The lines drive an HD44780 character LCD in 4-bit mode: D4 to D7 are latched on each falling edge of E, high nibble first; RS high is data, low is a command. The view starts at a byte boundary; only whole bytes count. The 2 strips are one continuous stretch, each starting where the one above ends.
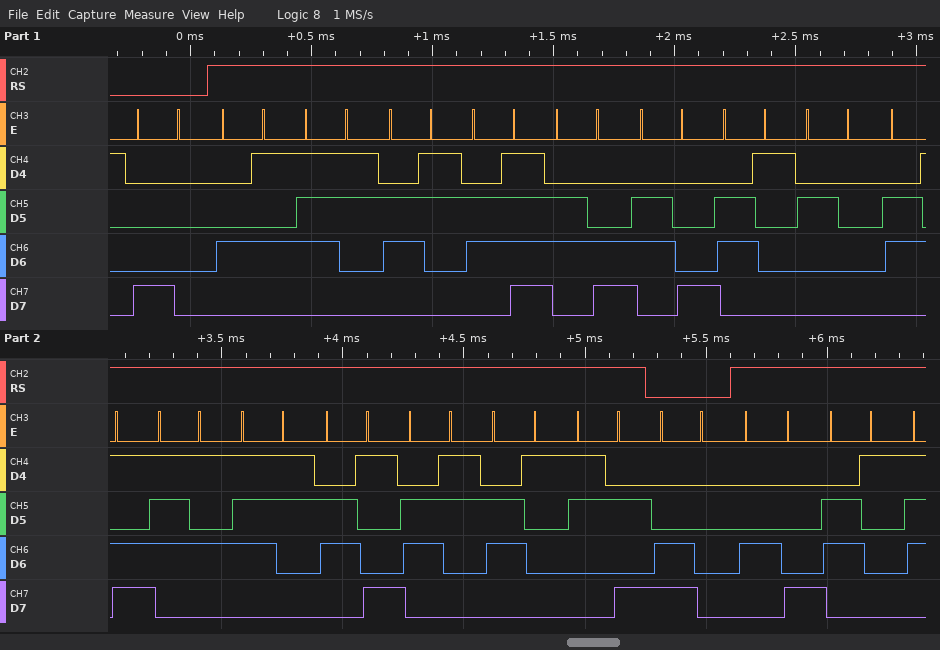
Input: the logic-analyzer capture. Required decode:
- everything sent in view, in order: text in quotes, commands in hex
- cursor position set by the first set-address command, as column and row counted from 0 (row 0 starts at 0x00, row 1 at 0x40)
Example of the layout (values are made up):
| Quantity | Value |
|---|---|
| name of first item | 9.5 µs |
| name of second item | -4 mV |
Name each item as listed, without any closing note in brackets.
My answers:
| Quantity | Value |
|---|---|
| everything sent in view, in order: text in quotes, commands in hex | 0x80 "Escolha musica:" 0xC0 "Ha" |
| cursor position set by the first set-address command, as column and row counted from 0 | column 0, row 0 |
